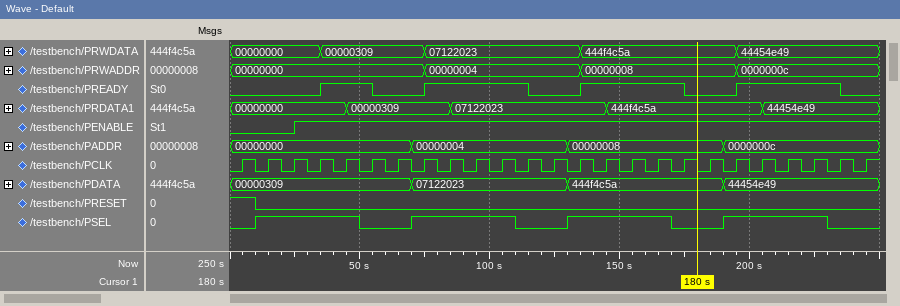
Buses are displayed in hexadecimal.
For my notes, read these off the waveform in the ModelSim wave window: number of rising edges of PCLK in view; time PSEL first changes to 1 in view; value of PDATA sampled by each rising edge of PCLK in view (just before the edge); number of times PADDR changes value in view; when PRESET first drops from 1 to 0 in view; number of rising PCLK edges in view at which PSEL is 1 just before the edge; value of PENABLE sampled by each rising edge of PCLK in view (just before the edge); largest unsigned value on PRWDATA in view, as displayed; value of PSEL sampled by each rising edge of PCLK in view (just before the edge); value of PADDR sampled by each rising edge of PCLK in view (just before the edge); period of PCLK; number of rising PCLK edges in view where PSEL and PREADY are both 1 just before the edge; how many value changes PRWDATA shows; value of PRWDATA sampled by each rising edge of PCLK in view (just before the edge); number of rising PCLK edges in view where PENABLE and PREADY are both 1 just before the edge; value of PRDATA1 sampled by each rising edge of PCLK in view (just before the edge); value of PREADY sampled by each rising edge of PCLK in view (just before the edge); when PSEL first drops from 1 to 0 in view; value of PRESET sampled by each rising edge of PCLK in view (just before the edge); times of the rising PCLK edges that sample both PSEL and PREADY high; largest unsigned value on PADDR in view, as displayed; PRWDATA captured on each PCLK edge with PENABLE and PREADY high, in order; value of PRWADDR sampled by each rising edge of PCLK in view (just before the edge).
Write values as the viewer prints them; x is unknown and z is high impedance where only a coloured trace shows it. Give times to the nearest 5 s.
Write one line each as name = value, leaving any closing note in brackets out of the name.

number of rising edges of PCLK in view = 25
time PSEL first changes to 1 in view = 10 s
value of PDATA sampled by each rising edge of PCLK in view = 00000309, 00000309, 00000309, 00000309, 00000309, 00000309, 00000309, 07122023, 07122023, 07122023, 07122023, 07122023, 07122023, 444f4c5a, 444f4c5a, 444f4c5a, 444f4c5a, 444f4c5a, 444f4c5a, 44454e49, 44454e49, 44454e49, 44454e49, 44454e49, 44454e49
number of times PADDR changes value in view = 3
when PRESET first drops from 1 to 0 in view = 10 s
number of rising PCLK edges in view at which PSEL is 1 just before the edge = 16
value of PENABLE sampled by each rising edge of PCLK in view = 0 0 0 1 1 1 1 1 1 1 1 1 1 1 1 1 1 1 1 1 1 1 1 1 1
largest unsigned value on PRWDATA in view, as displayed = 444f4c5a
value of PSEL sampled by each rising edge of PCLK in view = 0 1 1 1 1 0 0 1 1 1 1 0 0 1 1 1 1 0 0 1 1 1 1 0 0
value of PADDR sampled by each rising edge of PCLK in view = 00000000, 00000000, 00000000, 00000000, 00000000, 00000000, 00000000, 00000004, 00000004, 00000004, 00000004, 00000004, 00000004, 00000008, 00000008, 00000008, 00000008, 00000008, 00000008, 0000000c, 0000000c, 0000000c, 0000000c, 0000000c, 0000000c
period of PCLK = 10 s
number of rising PCLK edges in view where PSEL and PREADY are both 1 just before the edge = 10
how many value changes PRWDATA shows = 4
value of PRWDATA sampled by each rising edge of PCLK in view = 00000000, 00000000, 00000000, 00000000, 00000309, 00000309, 00000309, 00000309, 07122023, 07122023, 07122023, 07122023, 07122023, 07122023, 444f4c5a, 444f4c5a, 444f4c5a, 444f4c5a, 444f4c5a, 444f4c5a, 44454e49, 44454e49, 44454e49, 44454e49, 44454e49
number of rising PCLK edges in view where PENABLE and PREADY are both 1 just before the edge = 14
value of PRDATA1 sampled by each rising edge of PCLK in view = 00000000, 00000000, 00000000, 00000000, 00000000, 00000309, 00000309, 00000309, 00000309, 07122023, 07122023, 07122023, 07122023, 07122023, 07122023, 444f4c5a, 444f4c5a, 444f4c5a, 444f4c5a, 444f4c5a, 444f4c5a, 44454e49, 44454e49, 44454e49, 44454e49
value of PREADY sampled by each rising edge of PCLK in view = 0 0 0 0 1 1 0 0 1 1 1 1 0 0 1 1 1 1 0 0 1 1 1 1 0
when PSEL first drops from 1 to 0 in view = 50 s
value of PRESET sampled by each rising edge of PCLK in view = 1 0 0 0 0 0 0 0 0 0 0 0 0 0 0 0 0 0 0 0 0 0 0 0 0
times of the rising PCLK edges that sample both PSEL and PREADY high = 45 s, 85 s, 95 s, 105 s, 145 s, 155 s, 165 s, 205 s, 215 s, 225 s
largest unsigned value on PADDR in view, as displayed = 0000000c
PRWDATA captured on each PCLK edge with PENABLE and PREADY high, in order = 00000309, 00000309, 07122023, 07122023, 07122023, 07122023, 444f4c5a, 444f4c5a, 444f4c5a, 444f4c5a, 44454e49, 44454e49, 44454e49, 44454e49
value of PRWADDR sampled by each rising edge of PCLK in view = 00000000, 00000000, 00000000, 00000000, 00000000, 00000000, 00000000, 00000000, 00000004, 00000004, 00000004, 00000004, 00000004, 00000004, 00000008, 00000008, 00000008, 00000008, 00000008, 00000008, 0000000c, 0000000c, 0000000c, 0000000c, 0000000c
